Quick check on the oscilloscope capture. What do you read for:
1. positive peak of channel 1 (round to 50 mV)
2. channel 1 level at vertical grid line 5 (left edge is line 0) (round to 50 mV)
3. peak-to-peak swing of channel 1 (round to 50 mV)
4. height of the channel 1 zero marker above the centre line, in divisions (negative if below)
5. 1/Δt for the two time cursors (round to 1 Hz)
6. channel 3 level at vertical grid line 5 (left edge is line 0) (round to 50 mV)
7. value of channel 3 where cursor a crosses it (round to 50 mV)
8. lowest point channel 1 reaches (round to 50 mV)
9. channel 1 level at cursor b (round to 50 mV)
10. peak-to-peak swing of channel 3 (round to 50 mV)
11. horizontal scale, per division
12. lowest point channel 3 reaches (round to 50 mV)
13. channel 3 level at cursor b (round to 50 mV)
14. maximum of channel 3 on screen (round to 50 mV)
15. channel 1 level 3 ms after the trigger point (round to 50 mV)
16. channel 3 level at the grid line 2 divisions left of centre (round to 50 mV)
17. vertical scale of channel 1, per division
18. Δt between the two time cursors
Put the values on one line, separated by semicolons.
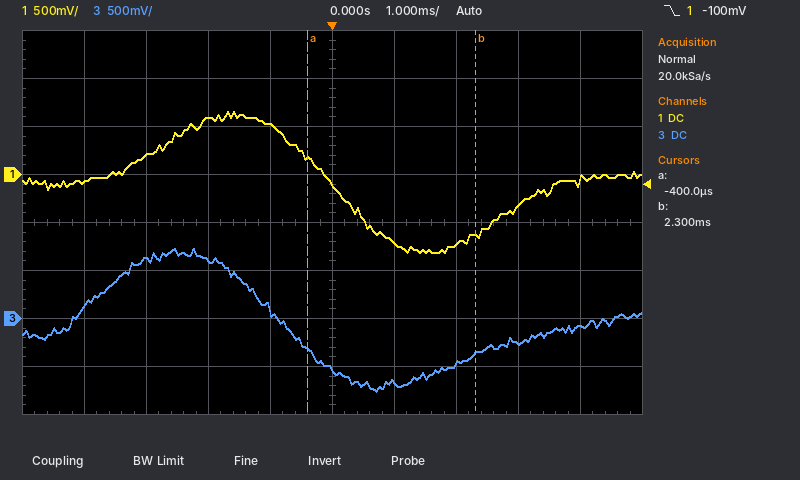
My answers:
650 mV; -100 mV; 1.45 V; +1.0 div; 370 Hz; -550 mV; -300 mV; -800 mV; -650 mV; 1.50 V; 1 ms; -750 mV; -350 mV; 750 mV; -350 mV; 600 mV; 500 mV; 2.7 ms
